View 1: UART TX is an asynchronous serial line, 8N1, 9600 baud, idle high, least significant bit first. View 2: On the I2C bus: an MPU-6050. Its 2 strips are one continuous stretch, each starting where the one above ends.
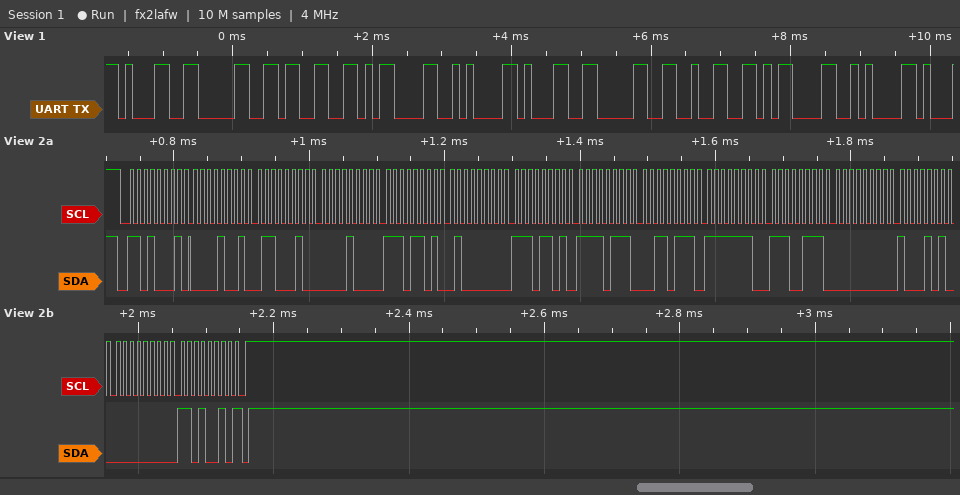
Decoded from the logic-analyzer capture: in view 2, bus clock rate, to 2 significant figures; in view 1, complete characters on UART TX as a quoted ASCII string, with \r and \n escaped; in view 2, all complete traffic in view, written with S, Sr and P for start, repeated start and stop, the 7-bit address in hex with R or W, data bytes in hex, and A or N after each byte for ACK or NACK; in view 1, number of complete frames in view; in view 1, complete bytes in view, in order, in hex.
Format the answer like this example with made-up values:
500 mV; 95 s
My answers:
100 kHz; "103\r\n102\r\n"; S 68R A 09 A 62 A 08 A ED A 40 A ED A F7 A 37 A FE A E7 A 00 A 8A A 00 A D2 N P; 10; 31 30 33 0D 0A 31 30 32 0D 0A
